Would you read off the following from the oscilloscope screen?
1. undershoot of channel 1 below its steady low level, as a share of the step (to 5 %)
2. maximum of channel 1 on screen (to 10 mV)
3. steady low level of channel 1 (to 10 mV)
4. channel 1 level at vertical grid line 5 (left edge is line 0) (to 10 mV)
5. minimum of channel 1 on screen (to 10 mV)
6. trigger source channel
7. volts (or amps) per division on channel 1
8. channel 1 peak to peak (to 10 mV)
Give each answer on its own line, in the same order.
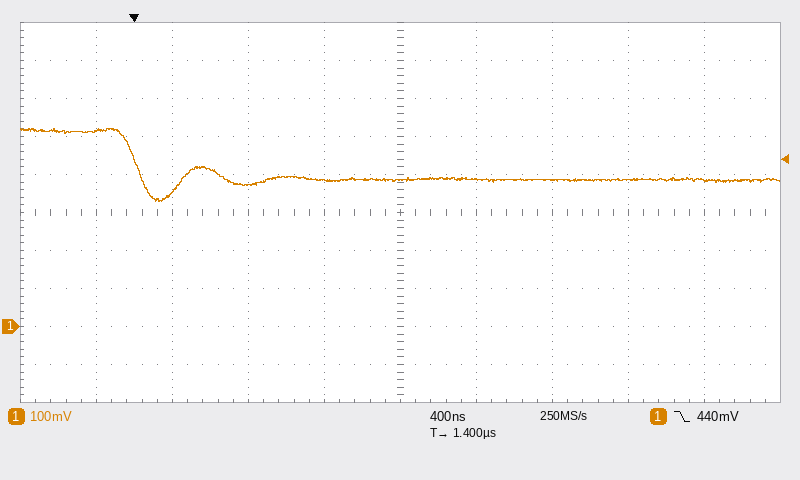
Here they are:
45 %
520 mV
390 mV
390 mV
330 mV
channel 1
100 mV
190 mV
